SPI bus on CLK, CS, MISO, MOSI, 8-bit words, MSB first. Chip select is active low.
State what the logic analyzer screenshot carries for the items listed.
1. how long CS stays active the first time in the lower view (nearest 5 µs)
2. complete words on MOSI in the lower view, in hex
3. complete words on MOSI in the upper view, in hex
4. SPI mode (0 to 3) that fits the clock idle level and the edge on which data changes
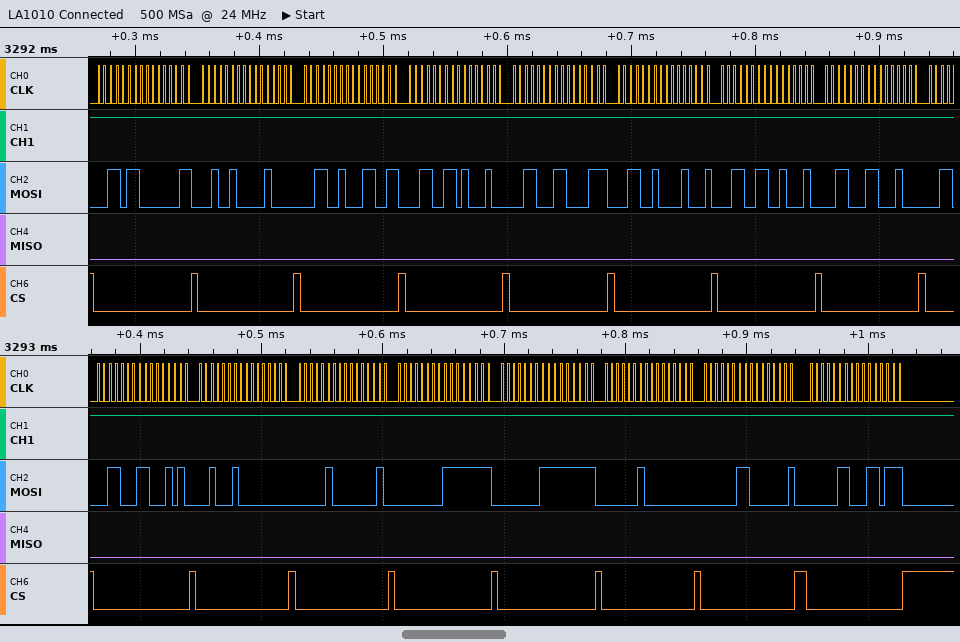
80 µs
31, 8A, 22, 00, 04, 02, 00, FF, 01, FF, 02, 00, 03, 01, 06, 37
36, 03, 24, 10, 32, 33, 33, 44, 31, 87, 32, 11, 33, 22, 31, 88
0
